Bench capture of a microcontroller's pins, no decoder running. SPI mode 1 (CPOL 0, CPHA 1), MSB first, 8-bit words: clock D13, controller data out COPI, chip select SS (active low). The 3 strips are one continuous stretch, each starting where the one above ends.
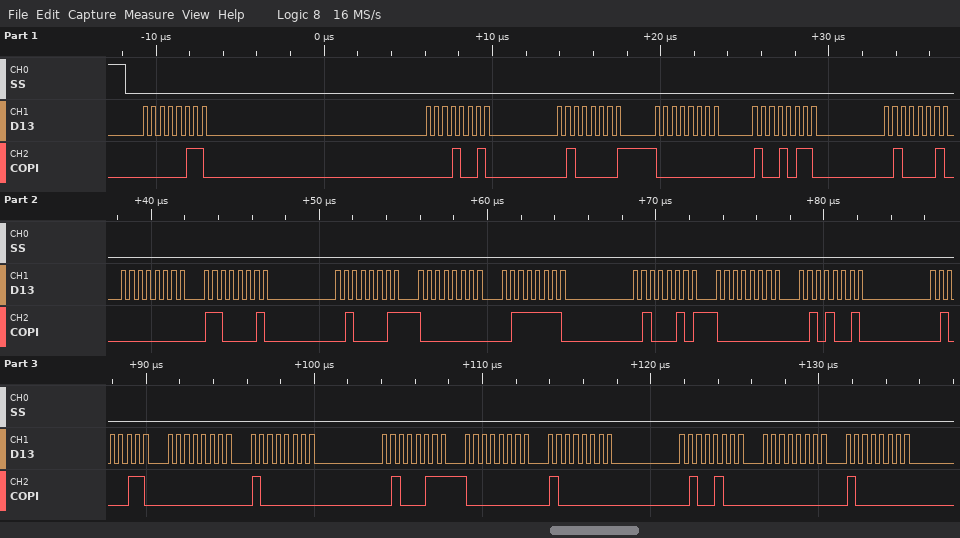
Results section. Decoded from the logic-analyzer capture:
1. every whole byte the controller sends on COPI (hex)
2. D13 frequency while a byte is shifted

06 12 41 00 96 42 00 C2 43 00 7E 45 00 52 46 00 80 47 00 80 48 00 80
2 MHz
